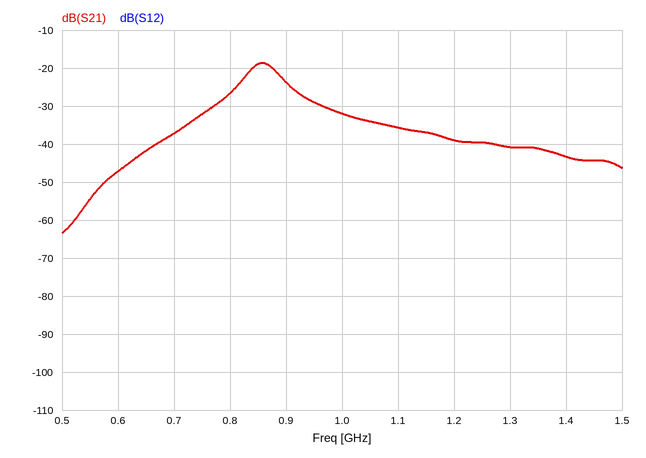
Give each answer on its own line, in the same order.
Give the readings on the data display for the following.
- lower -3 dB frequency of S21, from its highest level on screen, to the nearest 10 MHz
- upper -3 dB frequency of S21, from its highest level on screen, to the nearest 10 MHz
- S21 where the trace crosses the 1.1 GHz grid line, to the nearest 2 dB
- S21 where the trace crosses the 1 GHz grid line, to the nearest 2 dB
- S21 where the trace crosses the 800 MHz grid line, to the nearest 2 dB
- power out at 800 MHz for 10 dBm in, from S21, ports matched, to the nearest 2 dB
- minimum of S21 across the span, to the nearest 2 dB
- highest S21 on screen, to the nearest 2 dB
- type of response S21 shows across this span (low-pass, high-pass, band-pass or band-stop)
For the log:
830 MHz
890 MHz
-36 dB
-32 dB
-26 dB
-16 dBm
-64 dB
-18 dB
band-pass
